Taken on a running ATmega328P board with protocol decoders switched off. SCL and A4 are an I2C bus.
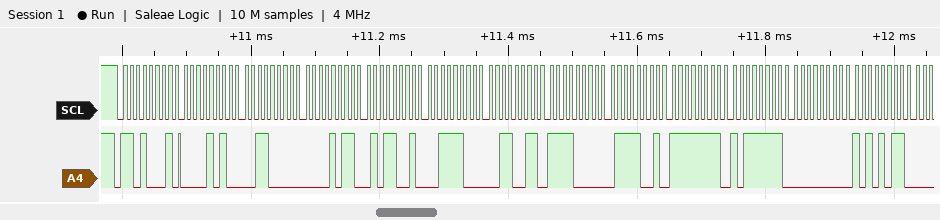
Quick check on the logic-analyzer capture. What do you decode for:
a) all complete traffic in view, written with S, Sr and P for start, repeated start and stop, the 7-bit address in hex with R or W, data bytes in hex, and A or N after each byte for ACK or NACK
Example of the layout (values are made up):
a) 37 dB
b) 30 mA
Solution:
a) S 68R A 0A A 30 A 0B A 59 A 3C A 33 A F0 A 79 A FF A BF A 00 A AB A
